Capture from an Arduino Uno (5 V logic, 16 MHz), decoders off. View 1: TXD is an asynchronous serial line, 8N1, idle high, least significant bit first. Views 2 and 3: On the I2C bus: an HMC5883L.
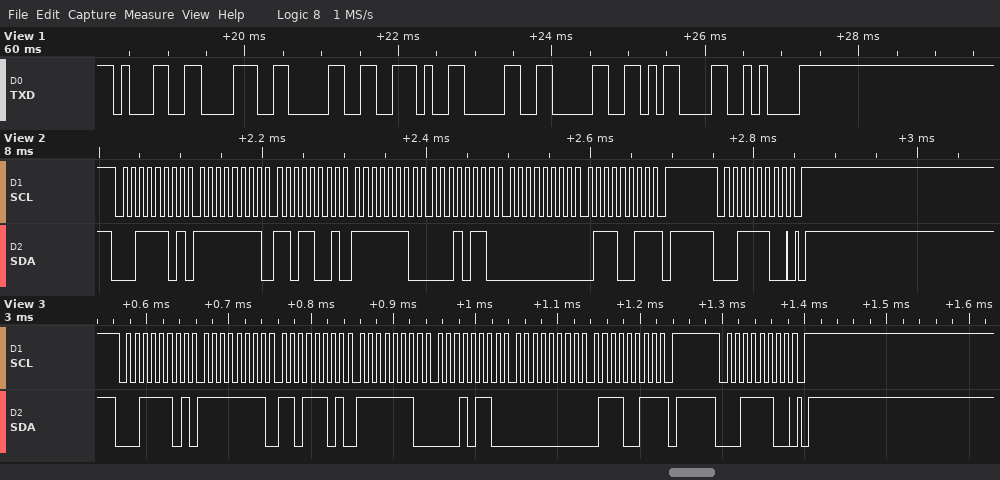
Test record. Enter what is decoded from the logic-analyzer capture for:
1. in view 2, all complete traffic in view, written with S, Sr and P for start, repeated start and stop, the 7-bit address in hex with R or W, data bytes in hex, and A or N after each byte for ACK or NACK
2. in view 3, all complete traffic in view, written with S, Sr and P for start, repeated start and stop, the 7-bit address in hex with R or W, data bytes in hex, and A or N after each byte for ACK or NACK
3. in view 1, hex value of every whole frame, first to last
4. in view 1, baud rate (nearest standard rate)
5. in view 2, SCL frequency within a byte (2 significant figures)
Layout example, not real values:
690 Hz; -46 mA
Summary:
S 1ER A FF A D9 A FE A 16 A 00 A 73 N P S 1EW A P; S 1ER A FF A DD A FE A 16 A 00 A 73 N P S 1EW A P; 31 38 30 2E 30 30 0D 0A; 9600 baud; 100 kHz
